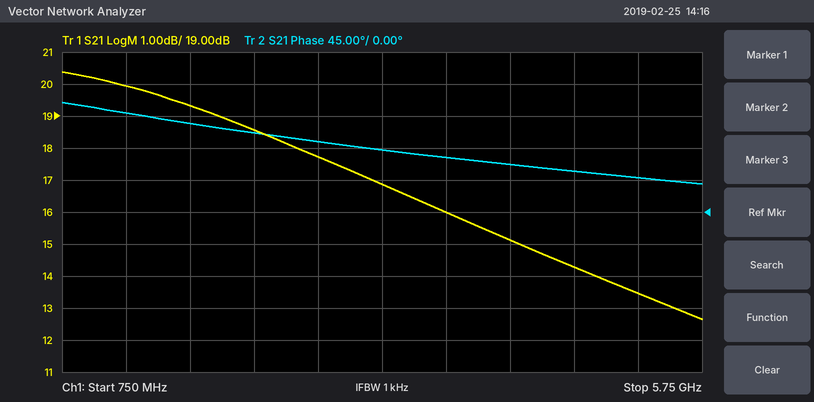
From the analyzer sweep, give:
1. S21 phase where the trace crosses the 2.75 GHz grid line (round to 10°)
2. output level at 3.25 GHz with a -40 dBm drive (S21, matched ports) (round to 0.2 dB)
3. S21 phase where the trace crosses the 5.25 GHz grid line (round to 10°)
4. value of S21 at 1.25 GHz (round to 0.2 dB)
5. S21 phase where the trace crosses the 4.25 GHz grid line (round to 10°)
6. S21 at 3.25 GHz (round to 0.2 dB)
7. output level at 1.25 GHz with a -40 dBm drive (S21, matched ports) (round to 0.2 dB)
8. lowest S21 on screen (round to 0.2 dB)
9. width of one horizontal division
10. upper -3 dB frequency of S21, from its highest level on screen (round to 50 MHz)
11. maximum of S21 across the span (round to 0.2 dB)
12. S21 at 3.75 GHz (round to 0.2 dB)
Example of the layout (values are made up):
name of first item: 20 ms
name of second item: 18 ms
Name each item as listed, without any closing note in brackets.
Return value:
S21 phase where the trace crosses the 2.75 GHz grid line: 100°
output level at 3.25 GHz with a -40 dBm drive (S21, matched ports): -23.2 dBm
S21 phase where the trace crosses the 5.25 GHz grid line: 50°
value of S21 at 1.25 GHz: 20.0 dB
S21 phase where the trace crosses the 4.25 GHz grid line: 70°
S21 at 3.25 GHz: 16.8 dB
output level at 1.25 GHz with a -40 dBm drive (S21, matched ports): -20.0 dBm
lowest S21 on screen: 12.6 dB
width of one horizontal division: 500 MHz
upper -3 dB frequency of S21, from its highest level on screen: 2.95 GHz
maximum of S21 across the span: 20.4 dB
S21 at 3.75 GHz: 16.0 dB
